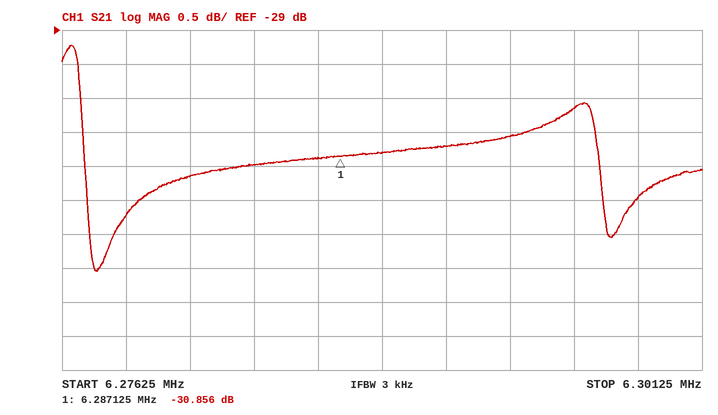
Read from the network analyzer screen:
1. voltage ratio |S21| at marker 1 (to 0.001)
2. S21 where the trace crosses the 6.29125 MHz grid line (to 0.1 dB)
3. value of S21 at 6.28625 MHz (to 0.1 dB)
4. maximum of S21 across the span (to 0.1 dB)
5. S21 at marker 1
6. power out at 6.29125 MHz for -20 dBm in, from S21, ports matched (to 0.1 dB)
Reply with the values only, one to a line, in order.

0.029
-30.7 dB
-30.9 dB
-29.2 dB
-30.856 dB
-50.7 dBm
